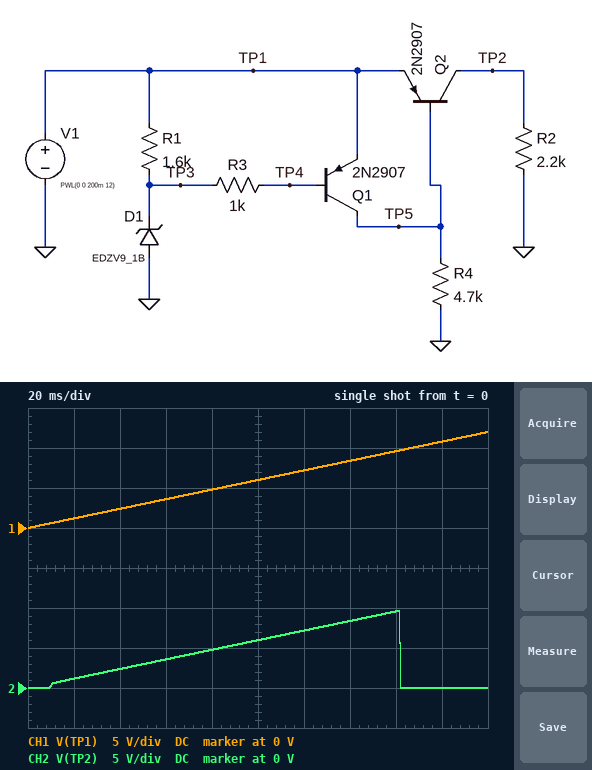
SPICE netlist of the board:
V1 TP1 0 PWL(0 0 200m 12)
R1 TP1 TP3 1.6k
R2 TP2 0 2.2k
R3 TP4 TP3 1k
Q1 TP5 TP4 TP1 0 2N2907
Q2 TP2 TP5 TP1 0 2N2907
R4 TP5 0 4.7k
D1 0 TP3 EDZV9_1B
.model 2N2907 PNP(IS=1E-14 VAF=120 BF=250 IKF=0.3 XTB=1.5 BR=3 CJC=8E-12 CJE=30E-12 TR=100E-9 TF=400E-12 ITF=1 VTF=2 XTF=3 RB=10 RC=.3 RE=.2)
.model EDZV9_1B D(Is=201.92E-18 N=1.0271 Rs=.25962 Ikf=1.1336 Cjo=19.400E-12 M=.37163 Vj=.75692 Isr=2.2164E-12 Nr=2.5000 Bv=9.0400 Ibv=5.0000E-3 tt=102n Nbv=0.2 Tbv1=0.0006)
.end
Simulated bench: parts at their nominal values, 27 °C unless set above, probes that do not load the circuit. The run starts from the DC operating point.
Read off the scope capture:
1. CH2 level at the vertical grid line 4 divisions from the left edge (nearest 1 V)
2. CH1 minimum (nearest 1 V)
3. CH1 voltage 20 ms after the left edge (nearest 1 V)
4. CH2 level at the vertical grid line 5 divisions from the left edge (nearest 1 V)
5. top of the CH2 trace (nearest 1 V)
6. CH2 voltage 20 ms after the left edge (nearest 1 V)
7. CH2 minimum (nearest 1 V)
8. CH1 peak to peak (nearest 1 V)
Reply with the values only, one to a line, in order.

5 V
0 V
1 V
6 V
10 V
1 V
0 V
12 V
